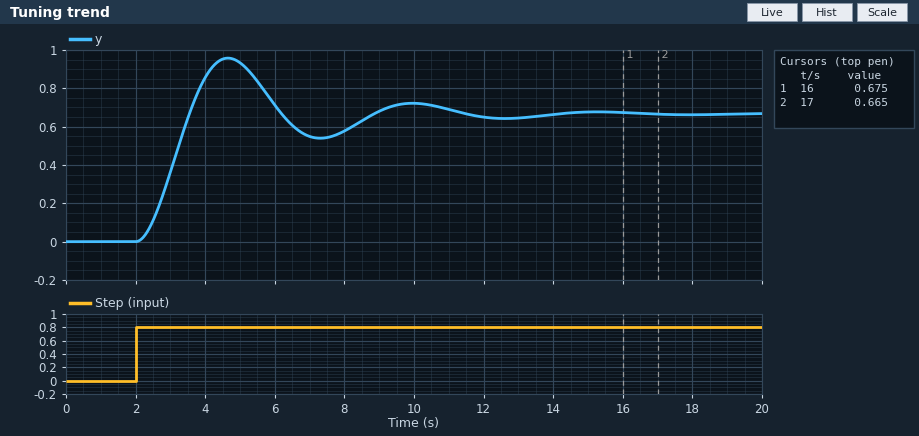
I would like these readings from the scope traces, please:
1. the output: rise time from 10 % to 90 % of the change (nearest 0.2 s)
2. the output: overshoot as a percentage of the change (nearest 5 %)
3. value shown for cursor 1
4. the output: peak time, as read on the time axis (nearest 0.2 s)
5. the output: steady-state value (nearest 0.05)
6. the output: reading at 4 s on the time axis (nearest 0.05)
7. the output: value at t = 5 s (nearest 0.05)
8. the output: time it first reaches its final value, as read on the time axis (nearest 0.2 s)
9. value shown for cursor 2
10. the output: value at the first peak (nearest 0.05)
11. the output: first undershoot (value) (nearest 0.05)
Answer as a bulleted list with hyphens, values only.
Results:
- 1.0 s
- 45 %
- 0.675
- 4.6 s
- 0.65
- 0.85
- 0.95
- 3.6 s
- 0.665
- 0.95
- 0.55
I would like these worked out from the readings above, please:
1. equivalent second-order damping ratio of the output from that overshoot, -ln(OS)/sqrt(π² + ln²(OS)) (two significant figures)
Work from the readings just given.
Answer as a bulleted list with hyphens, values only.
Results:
- 0.25
